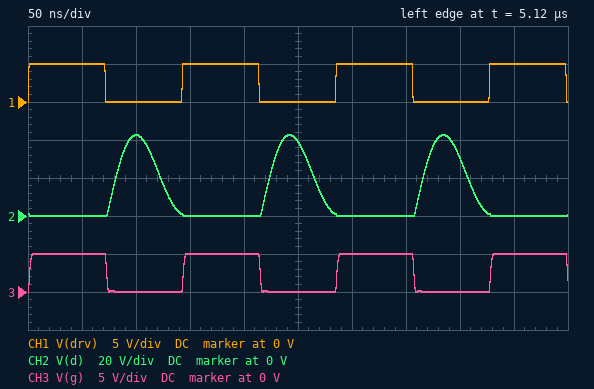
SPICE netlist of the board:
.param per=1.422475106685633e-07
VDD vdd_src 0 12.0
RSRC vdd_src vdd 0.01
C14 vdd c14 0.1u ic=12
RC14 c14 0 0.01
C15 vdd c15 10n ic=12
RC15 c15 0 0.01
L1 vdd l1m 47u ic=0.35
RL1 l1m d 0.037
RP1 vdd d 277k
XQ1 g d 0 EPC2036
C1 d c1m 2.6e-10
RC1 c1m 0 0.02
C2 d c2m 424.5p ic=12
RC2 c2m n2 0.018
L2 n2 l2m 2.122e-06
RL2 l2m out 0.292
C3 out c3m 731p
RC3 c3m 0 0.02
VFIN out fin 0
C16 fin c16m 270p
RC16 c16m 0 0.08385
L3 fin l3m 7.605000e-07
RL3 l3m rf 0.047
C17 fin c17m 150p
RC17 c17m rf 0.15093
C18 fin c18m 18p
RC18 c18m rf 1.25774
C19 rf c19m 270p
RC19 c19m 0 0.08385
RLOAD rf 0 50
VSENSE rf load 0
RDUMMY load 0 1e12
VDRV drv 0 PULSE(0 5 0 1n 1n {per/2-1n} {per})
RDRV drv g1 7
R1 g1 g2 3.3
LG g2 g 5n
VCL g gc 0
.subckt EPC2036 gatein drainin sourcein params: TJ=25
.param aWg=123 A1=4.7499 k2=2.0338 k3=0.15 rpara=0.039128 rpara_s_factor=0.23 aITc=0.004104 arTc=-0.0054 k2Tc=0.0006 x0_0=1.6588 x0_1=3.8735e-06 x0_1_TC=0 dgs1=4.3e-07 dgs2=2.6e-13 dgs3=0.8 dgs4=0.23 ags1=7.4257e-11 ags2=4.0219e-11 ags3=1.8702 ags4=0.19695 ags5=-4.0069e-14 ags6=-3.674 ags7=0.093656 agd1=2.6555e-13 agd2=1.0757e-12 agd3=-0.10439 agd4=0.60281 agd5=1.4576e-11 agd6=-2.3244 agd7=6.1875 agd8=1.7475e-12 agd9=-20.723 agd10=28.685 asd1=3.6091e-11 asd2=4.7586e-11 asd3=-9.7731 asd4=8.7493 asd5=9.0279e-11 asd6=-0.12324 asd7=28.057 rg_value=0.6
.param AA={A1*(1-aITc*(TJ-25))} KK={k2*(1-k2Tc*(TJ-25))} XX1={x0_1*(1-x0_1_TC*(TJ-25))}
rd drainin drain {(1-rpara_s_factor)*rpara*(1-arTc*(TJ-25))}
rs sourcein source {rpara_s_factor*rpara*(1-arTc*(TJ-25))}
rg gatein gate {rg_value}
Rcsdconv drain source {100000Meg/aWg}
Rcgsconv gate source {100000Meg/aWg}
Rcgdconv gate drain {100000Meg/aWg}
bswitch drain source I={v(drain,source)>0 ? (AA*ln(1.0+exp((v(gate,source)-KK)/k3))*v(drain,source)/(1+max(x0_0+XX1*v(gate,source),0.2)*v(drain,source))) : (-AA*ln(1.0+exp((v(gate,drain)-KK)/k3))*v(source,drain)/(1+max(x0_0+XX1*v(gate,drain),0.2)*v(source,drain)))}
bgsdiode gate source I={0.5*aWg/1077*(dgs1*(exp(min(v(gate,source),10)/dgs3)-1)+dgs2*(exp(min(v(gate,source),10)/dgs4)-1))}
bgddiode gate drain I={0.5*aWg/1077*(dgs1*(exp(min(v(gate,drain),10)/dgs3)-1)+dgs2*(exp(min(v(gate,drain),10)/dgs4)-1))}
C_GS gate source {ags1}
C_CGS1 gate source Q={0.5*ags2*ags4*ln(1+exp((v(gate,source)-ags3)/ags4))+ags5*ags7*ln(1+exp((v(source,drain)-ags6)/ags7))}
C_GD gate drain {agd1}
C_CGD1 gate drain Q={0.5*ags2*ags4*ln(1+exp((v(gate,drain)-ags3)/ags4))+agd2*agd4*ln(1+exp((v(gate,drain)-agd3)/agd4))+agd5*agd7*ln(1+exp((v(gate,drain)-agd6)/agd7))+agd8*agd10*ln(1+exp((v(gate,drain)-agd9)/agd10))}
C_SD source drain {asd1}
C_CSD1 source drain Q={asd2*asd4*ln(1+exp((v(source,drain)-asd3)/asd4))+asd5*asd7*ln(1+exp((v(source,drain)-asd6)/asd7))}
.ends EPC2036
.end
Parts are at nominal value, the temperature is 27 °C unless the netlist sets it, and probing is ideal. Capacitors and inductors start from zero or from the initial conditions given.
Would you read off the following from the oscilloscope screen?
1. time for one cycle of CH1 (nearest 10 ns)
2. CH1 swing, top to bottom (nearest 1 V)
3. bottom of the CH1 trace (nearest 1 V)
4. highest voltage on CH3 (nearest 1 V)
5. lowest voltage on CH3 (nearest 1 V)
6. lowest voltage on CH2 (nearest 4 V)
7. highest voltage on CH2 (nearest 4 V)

140 ns
5 V
0 V
5 V
0 V
0 V
44 V
